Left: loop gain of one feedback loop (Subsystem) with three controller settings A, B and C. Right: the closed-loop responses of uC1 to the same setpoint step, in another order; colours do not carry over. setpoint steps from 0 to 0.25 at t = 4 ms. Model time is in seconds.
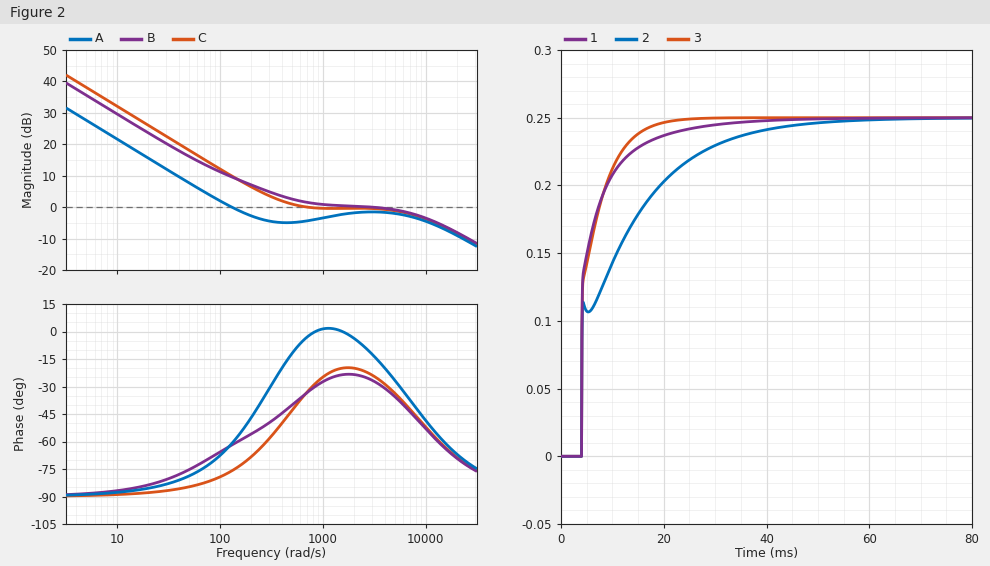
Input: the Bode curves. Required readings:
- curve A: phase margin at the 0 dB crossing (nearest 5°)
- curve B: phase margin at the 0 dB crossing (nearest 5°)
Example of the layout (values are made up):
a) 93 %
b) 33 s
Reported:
a) 120°
b) 155°
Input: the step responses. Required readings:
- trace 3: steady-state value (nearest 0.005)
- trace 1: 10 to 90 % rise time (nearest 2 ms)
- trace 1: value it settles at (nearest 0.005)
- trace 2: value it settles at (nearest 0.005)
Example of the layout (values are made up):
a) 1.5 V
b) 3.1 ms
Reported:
a) 0.250
b) 10 ms
c) 0.250
d) 0.250
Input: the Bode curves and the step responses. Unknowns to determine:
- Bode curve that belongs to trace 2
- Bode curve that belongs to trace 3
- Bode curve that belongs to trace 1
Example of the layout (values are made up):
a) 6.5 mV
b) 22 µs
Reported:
a) A
b) C
c) B
